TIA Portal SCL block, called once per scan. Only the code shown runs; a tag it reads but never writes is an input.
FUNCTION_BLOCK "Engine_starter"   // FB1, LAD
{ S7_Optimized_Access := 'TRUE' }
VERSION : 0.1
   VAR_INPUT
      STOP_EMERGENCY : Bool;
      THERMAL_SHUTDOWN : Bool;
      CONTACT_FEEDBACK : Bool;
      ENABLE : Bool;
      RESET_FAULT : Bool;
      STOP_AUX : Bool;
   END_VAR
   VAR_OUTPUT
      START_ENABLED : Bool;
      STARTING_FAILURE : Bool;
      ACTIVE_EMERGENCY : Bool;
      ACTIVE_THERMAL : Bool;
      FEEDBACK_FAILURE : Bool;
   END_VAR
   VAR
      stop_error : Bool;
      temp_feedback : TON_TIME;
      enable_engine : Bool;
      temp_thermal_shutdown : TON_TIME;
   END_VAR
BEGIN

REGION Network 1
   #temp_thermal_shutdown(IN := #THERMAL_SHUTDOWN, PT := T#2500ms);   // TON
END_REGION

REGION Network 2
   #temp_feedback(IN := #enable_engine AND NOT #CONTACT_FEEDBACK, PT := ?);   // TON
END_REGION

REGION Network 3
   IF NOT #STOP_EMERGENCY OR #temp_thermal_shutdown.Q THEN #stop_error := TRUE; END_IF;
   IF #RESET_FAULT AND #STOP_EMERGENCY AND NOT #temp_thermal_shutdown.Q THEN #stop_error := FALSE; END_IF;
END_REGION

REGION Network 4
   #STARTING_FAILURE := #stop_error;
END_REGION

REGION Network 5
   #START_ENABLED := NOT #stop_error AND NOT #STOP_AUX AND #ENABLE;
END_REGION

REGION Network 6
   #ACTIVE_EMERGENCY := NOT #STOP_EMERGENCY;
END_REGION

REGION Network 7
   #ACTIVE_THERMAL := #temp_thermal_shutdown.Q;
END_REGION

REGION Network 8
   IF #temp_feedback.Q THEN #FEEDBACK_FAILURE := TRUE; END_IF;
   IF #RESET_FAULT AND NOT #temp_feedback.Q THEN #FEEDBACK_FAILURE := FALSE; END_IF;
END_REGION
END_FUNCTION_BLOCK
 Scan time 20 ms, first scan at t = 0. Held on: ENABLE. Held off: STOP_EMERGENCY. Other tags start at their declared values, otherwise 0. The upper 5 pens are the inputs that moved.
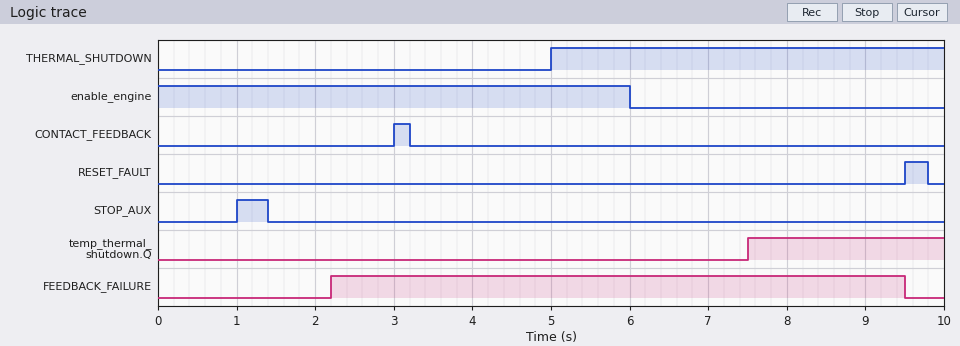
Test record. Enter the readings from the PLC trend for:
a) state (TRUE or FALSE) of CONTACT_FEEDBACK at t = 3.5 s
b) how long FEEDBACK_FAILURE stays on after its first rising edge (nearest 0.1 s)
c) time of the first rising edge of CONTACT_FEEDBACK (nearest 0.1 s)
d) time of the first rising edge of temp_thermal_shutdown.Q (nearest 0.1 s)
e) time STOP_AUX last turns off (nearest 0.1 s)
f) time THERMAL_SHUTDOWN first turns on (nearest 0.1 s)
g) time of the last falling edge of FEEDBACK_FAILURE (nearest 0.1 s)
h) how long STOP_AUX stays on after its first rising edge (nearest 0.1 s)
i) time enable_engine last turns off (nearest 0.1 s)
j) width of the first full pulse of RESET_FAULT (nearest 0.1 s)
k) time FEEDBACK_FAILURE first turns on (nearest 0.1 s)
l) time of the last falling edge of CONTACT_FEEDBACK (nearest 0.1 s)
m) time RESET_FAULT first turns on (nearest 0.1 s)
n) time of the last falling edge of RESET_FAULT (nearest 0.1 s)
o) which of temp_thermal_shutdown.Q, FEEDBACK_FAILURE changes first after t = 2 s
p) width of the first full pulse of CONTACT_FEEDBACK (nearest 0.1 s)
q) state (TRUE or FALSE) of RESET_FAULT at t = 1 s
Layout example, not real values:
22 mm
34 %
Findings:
FALSE
7.3 s
3.0 s
7.5 s
1.4 s
5.0 s
9.5 s
0.4 s
6.0 s
0.3 s
2.2 s
3.2 s
9.5 s
9.8 s
FEEDBACK_FAILURE
0.2 s
FALSE
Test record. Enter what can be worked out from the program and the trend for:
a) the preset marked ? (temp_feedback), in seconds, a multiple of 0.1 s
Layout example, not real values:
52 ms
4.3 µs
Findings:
2.2 s
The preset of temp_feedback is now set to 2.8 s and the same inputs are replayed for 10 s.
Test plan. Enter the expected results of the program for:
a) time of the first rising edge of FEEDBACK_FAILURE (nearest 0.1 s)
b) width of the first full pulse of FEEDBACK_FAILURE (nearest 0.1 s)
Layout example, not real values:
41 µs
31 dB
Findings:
2.8 s
6.7 s
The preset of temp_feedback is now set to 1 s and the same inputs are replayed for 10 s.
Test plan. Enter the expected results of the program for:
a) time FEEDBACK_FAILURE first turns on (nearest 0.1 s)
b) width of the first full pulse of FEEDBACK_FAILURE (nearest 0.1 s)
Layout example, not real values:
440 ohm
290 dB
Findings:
1.0 s
8.5 s
